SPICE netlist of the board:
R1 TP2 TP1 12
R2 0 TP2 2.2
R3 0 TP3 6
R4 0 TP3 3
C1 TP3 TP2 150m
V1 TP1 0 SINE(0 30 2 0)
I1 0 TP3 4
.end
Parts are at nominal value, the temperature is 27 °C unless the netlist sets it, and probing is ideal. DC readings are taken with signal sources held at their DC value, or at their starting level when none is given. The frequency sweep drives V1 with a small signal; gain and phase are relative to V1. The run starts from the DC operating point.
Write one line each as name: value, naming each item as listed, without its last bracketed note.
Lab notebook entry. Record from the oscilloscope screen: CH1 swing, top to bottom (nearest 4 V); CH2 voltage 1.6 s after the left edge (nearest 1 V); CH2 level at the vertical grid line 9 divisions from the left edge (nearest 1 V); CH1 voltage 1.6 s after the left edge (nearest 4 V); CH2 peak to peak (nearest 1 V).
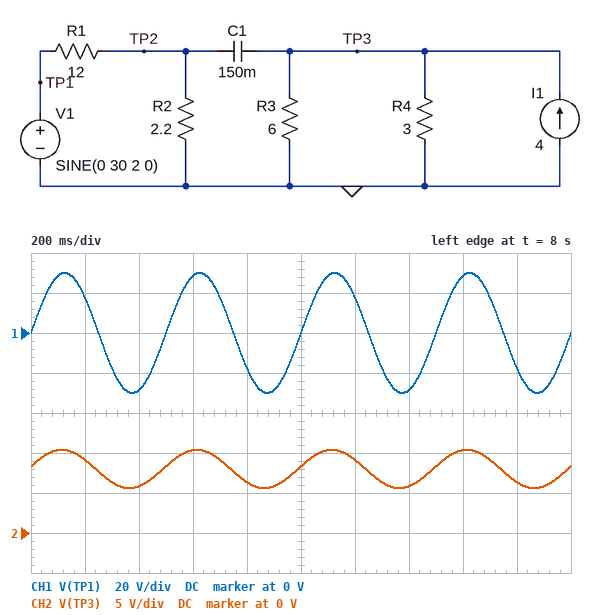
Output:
CH1 swing, top to bottom: 60 V
CH2 voltage 1.6 s after the left edge: 10 V
CH2 level at the vertical grid line 9 divisions from the left edge: 6 V
CH1 voltage 1.6 s after the left edge: 28 V
CH2 peak to peak: 5 V
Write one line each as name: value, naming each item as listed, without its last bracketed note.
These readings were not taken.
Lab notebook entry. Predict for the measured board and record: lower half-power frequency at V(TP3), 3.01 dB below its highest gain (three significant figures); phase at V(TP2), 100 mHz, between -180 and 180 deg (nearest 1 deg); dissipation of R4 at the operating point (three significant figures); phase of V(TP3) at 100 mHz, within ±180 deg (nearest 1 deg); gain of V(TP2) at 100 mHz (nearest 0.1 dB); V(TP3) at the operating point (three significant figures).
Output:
lower half-power frequency at V(TP3), 3.01 dB below its highest gain: 275 mHz
phase at V(TP2), 100 mHz, between -180 and 180 deg: -9 deg
dissipation of R4 at the operating point: 21.3 W
phase of V(TP3) at 100 mHz, within ±180 deg: 70 deg
gain of V(TP2) at 100 mHz: -16.6 dB
V(TP3) at the operating point: 8.00 V
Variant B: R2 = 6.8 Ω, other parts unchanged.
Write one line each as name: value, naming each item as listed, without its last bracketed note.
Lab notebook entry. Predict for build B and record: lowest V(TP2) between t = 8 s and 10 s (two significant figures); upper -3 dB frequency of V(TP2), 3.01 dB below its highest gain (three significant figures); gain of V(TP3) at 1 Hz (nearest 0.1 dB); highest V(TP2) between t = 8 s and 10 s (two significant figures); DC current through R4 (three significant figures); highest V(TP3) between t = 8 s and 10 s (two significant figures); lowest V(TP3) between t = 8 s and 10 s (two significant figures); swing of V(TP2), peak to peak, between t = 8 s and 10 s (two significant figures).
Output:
lowest V(TP2) between t = 8 s and 10 s: -3.5 V
upper -3 dB frequency of V(TP2), 3.01 dB below its highest gain: 187 mHz
gain of V(TP3) at 1 Hz: -19.0 dB
highest V(TP2) between t = 8 s and 10 s: 3.5 V
DC current through R4: 2.67 A
highest V(TP3) between t = 8 s and 10 s: 11 V
lowest V(TP3) between t = 8 s and 10 s: 4.6 V
swing of V(TP2), peak to peak, between t = 8 s and 10 s: 7.1 V
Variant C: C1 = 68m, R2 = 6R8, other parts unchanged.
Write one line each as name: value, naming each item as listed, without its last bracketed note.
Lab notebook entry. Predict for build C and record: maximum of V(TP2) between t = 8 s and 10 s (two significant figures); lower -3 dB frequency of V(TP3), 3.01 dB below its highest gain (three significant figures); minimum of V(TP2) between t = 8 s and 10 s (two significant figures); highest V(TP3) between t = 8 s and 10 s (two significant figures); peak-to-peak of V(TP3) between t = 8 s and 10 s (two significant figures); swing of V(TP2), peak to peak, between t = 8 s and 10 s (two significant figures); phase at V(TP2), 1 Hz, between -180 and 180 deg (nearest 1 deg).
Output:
maximum of V(TP2) between t = 8 s and 10 s: 3.9 V
lower -3 dB frequency of V(TP3), 3.01 dB below its highest gain: 369 mHz
minimum of V(TP2) between t = 8 s and 10 s: -3.9 V
highest V(TP3) between t = 8 s and 10 s: 11 V
peak-to-peak of V(TP3) between t = 8 s and 10 s: 6.7 V
swing of V(TP2), peak to peak, between t = 8 s and 10 s: 7.8 V
phase at V(TP2), 1 Hz, between -180 and 180 deg: -29 deg
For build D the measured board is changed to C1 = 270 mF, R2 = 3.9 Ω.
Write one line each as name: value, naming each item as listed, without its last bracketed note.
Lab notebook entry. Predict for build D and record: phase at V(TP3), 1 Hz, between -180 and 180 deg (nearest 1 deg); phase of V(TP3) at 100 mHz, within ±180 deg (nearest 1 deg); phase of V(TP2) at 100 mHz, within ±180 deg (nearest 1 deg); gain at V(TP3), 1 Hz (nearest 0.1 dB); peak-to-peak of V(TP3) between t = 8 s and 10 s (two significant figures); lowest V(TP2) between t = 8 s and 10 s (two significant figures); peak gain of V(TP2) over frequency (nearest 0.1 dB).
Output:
phase at V(TP3), 1 Hz, between -180 and 180 deg: 7 deg
phase of V(TP3) at 100 mHz, within ±180 deg: 50 deg
phase of V(TP2) at 100 mHz, within ±180 deg: -21 deg
gain at V(TP3), 1 Hz: -20.1 dB
peak-to-peak of V(TP3) between t = 8 s and 10 s: 5.9 V
lowest V(TP2) between t = 8 s and 10 s: -3.0 V
peak gain of V(TP2) over frequency: -12.2 dB
